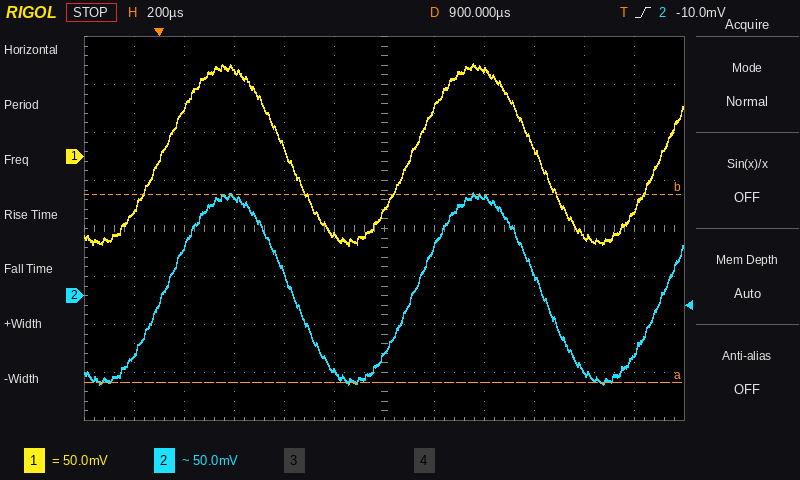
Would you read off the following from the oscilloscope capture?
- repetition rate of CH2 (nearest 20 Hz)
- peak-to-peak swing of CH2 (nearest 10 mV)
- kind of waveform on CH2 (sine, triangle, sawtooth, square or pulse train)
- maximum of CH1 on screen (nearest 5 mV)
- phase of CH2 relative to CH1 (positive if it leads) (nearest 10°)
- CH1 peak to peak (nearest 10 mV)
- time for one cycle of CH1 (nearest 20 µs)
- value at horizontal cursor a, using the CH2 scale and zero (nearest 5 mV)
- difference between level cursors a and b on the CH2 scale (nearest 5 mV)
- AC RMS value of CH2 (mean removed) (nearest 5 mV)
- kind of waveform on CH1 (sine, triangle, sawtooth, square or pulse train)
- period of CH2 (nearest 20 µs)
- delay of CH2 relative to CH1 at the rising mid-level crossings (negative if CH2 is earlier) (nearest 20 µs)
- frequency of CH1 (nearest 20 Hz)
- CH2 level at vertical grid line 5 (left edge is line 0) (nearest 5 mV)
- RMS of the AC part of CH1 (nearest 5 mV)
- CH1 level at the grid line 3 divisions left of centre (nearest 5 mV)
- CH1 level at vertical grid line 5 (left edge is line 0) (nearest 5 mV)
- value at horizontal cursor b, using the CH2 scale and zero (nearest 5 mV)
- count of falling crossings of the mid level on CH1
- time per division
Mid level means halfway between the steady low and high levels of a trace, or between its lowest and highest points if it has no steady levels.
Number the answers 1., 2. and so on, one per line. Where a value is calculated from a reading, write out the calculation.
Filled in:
1. 1 / 1.00 ms ≈ 1.00 kHz
2. 200 mV
3. sine
4. 95 mV
5. −360° × (+20 µs) / 1.00 ms ≈ -7.20°, so -10° to the nearest 10°
6. 190 mV
7. 1.00 ms
8. -90 mV
9. 195 mV
10. 200 mV / (2√2) ≈ 70.7 mV, so 70 mV to the nearest 5 mV
11. sine
12. 1.00 ms
13. +20 µs
14. 1 / 1.00 ms ≈ 1.00 kHz
15. -80 mV
16. 190 mV / (2√2) ≈ 67.2 mV, so 65 mV to the nearest 5 mV
17. 90 mV
18. -80 mV
19. 105 mV
20. 2
21. 200 µs
